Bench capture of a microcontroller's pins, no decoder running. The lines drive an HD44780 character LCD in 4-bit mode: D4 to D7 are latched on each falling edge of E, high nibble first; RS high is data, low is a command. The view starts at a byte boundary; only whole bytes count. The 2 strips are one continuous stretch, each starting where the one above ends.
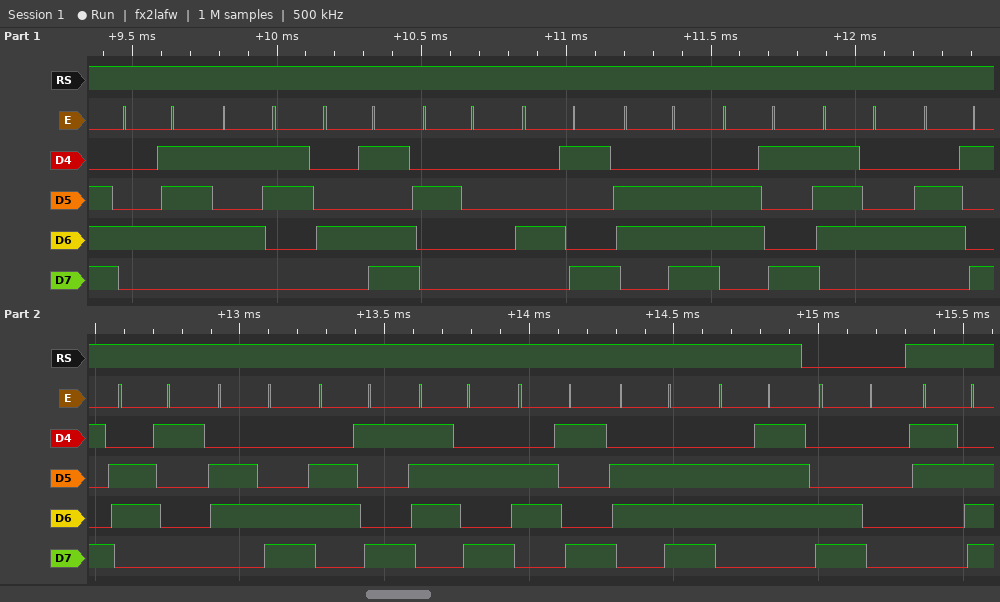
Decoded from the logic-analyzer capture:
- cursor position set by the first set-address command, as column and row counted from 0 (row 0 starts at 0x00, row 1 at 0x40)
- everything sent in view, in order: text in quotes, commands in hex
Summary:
column 0, row 1
"GSM Initializing" 0xC0 ">"
